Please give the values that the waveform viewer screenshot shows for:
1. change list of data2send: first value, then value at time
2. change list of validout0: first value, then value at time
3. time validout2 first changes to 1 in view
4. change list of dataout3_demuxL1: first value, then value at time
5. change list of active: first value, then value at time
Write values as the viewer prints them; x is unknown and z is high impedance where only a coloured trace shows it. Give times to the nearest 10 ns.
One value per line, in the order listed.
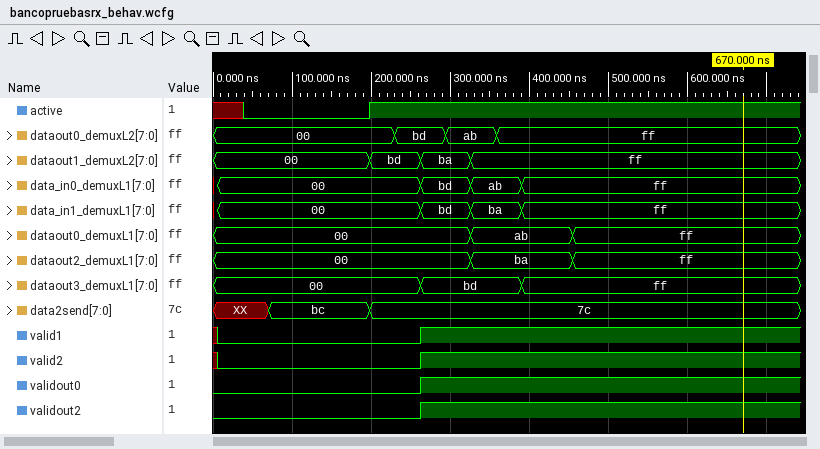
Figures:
XX, bc at 70 ns, 7c at 200 ns
0, 1 at 260 ns
260 ns
00, bd at 260 ns, ff at 390 ns
x, 0 at 40 ns, 1 at 200 ns
